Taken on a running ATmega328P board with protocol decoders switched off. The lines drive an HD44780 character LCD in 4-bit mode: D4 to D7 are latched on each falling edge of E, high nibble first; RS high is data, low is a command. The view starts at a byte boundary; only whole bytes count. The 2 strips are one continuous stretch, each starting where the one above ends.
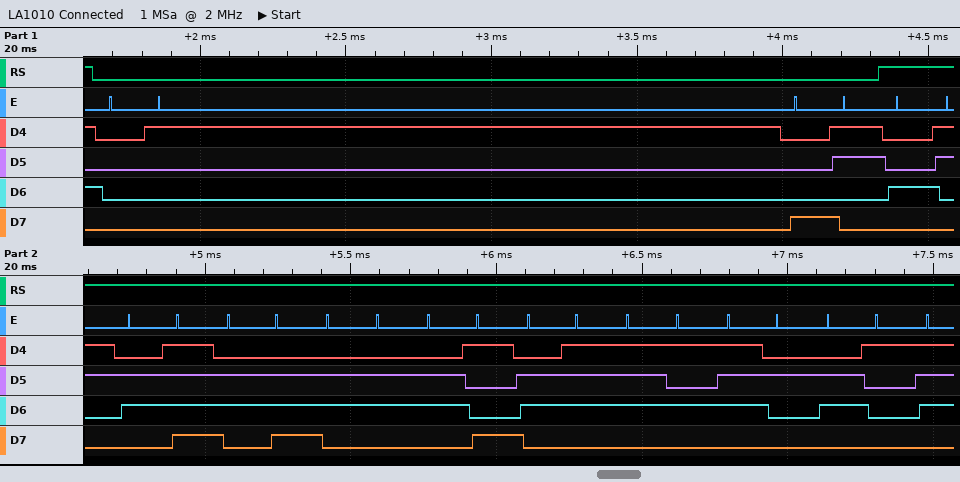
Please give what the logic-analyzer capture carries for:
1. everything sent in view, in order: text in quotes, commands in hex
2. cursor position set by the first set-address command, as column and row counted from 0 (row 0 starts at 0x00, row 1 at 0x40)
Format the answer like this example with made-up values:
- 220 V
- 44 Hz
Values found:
- 0x01 0x83 "Configura"
- column 3, row 0
